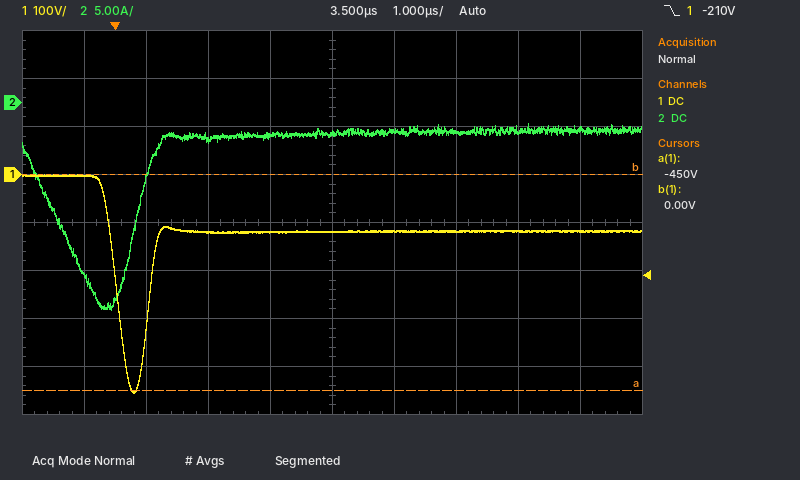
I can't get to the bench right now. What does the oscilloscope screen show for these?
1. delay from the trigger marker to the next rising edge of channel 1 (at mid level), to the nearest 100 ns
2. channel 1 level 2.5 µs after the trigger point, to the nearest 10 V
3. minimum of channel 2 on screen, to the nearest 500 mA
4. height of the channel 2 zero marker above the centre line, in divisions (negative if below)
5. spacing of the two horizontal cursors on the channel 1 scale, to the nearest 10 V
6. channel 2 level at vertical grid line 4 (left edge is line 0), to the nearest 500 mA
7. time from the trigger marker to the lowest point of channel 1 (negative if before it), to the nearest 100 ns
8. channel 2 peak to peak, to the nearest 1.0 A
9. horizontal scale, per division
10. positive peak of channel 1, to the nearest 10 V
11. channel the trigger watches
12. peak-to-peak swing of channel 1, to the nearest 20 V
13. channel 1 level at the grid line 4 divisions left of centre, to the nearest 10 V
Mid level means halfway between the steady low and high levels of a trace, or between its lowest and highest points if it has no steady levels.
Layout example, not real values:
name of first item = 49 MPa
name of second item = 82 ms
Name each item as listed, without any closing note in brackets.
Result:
delay from the trigger marker to the next rising edge of channel 1 (at mid level), to the nearest 100 ns = 600 ns
channel 1 level 2.5 µs after the trigger point, to the nearest 10 V = -120 V
minimum of channel 2 on screen, to the nearest 500 mA = -21.5 A
height of the channel 2 zero marker above the centre line, in divisions = +2.5 div
spacing of the two horizontal cursors on the channel 1 scale, to the nearest 10 V = 450 V
channel 2 level at vertical grid line 4 (left edge is line 0), to the nearest 500 mA = -3.5 A
time from the trigger marker to the lowest point of channel 1 (negative if before it), to the nearest 100 ns = +300 ns
channel 2 peak to peak, to the nearest 1.0 A = 19.0 A
horizontal scale, per division = 1 µs
positive peak of channel 1, to the nearest 10 V = 0 V
channel the trigger watches = channel 1
peak-to-peak swing of channel 1, to the nearest 20 V = 460 V
channel 1 level at the grid line 4 divisions left of centre, to the nearest 10 V = 0 V
